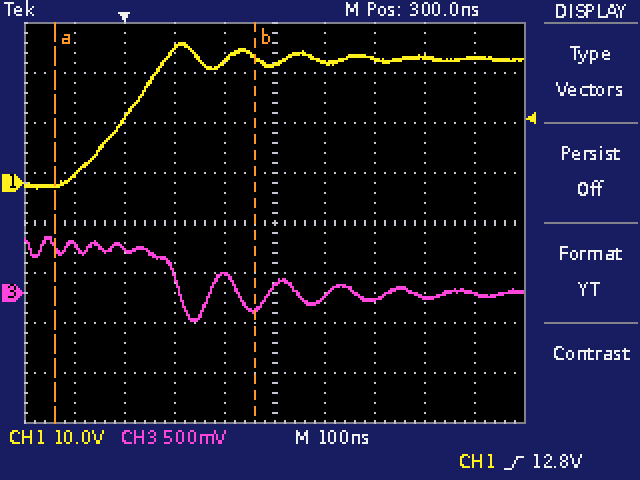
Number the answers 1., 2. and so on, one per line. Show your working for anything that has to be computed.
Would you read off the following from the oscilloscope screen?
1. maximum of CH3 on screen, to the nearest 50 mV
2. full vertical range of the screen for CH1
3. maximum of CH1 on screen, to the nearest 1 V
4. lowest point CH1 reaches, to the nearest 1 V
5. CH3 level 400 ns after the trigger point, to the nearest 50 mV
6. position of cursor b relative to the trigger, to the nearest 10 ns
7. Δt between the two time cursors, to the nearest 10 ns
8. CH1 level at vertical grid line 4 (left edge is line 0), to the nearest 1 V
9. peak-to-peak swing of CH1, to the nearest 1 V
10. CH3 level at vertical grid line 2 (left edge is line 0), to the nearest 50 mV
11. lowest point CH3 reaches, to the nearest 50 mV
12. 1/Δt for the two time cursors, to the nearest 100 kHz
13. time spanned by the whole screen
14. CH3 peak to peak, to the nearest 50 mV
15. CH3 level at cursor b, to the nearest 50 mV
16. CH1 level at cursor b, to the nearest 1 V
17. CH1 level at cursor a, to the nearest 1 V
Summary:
1. 550 mV
2. 80 V
3. 28 V
4. -1 V
5. -50 mV
6. +260 ns
7. 400 ns
8. 24 V
9. 28 V − (-1 V) = 29 V
10. 450 mV
11. -300 mV
12. 1 / 400 ns ≈ 2.5 MHz
13. 1 µs
14. 550 mV − (-300 mV) = 850 mV
15. -150 mV
16. 25 V
17. 0 V
